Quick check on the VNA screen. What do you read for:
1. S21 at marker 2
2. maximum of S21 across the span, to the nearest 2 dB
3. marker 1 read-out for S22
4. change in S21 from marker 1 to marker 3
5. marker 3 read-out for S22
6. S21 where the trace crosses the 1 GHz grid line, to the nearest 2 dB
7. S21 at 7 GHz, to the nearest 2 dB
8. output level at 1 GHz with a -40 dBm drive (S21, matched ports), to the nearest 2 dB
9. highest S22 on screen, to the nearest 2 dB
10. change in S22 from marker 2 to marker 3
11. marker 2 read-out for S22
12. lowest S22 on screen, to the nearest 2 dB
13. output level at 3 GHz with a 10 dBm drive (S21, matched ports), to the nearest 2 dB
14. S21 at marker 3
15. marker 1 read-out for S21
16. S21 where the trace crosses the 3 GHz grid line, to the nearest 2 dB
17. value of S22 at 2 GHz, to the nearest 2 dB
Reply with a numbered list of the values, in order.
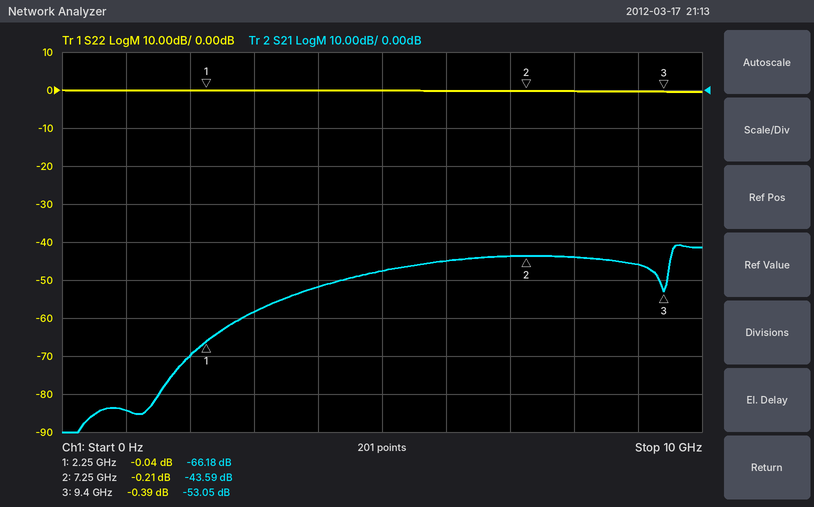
1. -43.59 dB
2. -40 dB
3. -0.04 dB
4. 13.13 dB
5. -0.39 dB
6. -84 dB
7. -44 dB
8. -124 dBm
9. 0 dB
10. -0.18 dB
11. -0.21 dB
12. 0 dB
13. -48 dBm
14. -53.05 dB
15. -66.18 dB
16. -58 dB
17. 0 dB
